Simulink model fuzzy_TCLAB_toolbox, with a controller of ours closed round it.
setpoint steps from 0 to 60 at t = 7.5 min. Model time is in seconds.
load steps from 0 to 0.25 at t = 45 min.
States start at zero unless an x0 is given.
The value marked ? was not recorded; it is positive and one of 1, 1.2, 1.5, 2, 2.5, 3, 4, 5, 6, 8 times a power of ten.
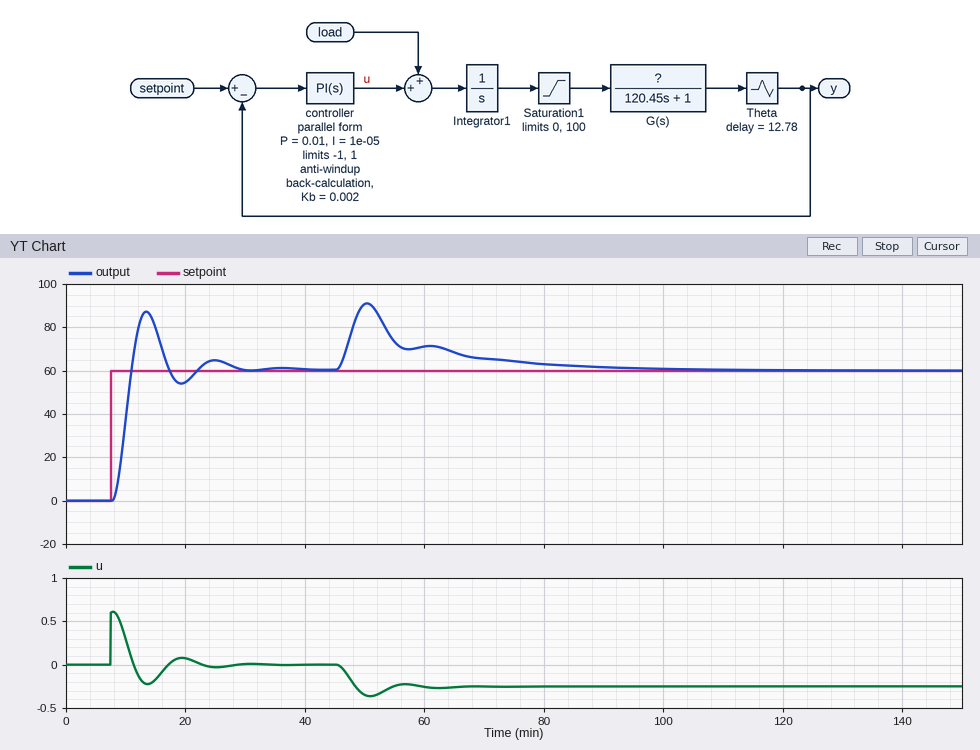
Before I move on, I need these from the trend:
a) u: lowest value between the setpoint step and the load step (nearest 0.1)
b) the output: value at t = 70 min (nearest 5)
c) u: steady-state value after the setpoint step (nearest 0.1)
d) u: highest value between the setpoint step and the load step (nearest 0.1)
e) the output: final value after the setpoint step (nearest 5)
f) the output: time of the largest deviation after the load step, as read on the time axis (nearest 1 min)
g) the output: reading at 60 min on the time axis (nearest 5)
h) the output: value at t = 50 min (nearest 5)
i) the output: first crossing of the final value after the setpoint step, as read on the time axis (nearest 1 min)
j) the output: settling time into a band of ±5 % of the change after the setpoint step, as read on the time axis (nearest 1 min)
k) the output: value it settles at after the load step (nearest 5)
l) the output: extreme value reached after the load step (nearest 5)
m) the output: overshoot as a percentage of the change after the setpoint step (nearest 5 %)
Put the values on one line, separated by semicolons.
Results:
-0.2; 65; 0.0; 0.6; 60; 50 min; 70; 90; 11 min; 27 min; 60; 90; 45 %
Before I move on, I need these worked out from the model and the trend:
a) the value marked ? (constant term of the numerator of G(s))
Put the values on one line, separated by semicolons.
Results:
1.2
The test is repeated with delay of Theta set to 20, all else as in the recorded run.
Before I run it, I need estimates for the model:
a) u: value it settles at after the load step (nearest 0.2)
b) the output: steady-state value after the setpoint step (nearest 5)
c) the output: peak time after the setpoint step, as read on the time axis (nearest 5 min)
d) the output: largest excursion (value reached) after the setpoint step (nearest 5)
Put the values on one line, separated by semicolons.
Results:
-0.2; 60; 15 min; 90
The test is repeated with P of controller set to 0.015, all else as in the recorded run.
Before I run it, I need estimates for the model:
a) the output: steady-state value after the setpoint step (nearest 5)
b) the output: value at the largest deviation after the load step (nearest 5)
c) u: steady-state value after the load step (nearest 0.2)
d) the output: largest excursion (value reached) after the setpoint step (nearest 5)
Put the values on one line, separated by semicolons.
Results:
60; 85; -0.2; 90
